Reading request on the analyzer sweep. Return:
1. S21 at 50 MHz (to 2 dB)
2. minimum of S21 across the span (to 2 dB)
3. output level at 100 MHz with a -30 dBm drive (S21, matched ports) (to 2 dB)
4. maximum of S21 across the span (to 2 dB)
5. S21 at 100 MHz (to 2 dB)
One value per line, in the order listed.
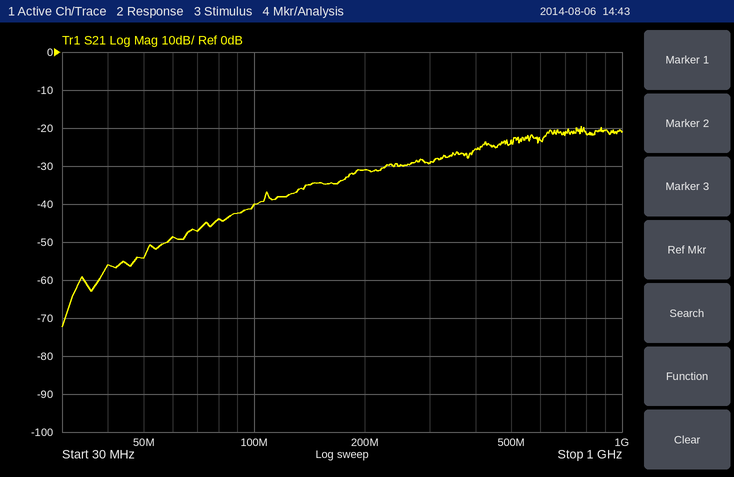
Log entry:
-54 dB
-72 dB
-70 dBm
-20 dB
-40 dB
